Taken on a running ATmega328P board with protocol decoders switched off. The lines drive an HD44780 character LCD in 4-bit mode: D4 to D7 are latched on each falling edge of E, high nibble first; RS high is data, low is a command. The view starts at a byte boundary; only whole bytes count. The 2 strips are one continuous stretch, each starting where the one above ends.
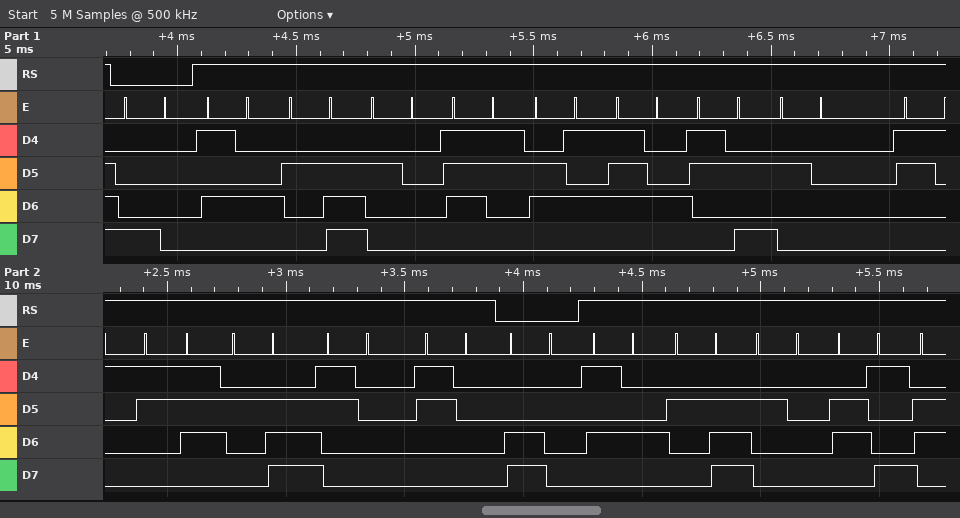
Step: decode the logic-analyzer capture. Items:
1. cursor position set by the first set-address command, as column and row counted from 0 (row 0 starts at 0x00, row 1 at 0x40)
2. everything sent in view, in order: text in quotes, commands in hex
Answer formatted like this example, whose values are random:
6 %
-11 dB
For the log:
column 0, row 0
0x80 "T. set: 17.00" 0xC0 "T. i"
